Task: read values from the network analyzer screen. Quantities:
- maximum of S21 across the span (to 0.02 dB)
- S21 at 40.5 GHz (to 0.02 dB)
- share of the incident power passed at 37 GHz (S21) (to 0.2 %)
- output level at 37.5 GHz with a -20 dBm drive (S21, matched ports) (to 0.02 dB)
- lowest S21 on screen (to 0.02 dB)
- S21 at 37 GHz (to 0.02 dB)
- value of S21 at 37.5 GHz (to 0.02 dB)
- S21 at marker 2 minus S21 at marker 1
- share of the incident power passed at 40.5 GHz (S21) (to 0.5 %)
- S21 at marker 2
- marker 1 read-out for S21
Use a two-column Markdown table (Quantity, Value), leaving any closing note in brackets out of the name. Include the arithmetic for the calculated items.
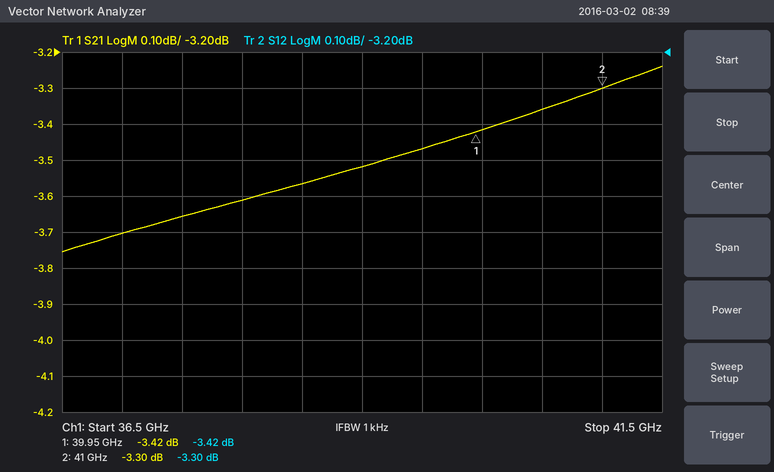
| Quantity | Value |
|---|---|
| maximum of S21 across the span | -3.24 dB |
| S21 at 40.5 GHz | -3.36 dB |
| share of the incident power passed at 37 GHz (S21) | 10^(-3.7/10) ≈ 42.7 %, so 42.6 % to the nearest 0.2 % |
| output level at 37.5 GHz with a -20 dBm drive (S21, matched ports) | -20 dBm + (-3.66 dB) = -23.66 dBm |
| lowest S21 on screen | -3.76 dB |
| S21 at 37 GHz | -3.70 dB |
| value of S21 at 37.5 GHz | -3.66 dB |
| S21 at marker 2 minus S21 at marker 1 | -3.3 − (-3.42) = 0.12 dB |
| share of the incident power passed at 40.5 GHz (S21) | 10^(-3.36/10) ≈ 46.1 %, so 46.0 % to the nearest 0.5 % |
| S21 at marker 2 | -3.30 dB |
| marker 1 read-out for S21 | -3.42 dB |
